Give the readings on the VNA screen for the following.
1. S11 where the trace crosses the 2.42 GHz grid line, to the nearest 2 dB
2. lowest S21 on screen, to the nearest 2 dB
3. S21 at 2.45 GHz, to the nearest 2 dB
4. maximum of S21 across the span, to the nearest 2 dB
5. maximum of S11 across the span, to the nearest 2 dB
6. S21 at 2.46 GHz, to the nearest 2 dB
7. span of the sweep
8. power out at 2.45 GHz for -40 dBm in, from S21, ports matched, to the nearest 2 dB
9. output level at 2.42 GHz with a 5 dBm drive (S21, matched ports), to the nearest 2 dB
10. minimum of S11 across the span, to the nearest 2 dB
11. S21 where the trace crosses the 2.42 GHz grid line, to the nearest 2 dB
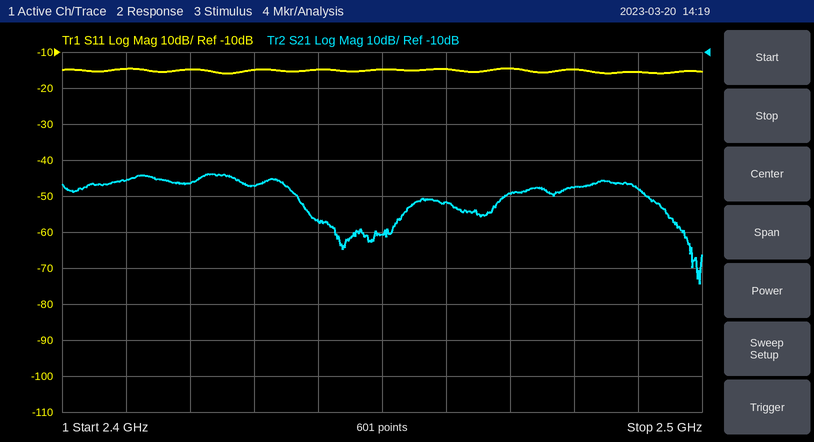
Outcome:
-14 dB
-74 dB
-60 dB
-44 dB
-14 dB
-52 dB
100 MHz
-100 dBm
-42 dBm
-16 dB
-46 dB
